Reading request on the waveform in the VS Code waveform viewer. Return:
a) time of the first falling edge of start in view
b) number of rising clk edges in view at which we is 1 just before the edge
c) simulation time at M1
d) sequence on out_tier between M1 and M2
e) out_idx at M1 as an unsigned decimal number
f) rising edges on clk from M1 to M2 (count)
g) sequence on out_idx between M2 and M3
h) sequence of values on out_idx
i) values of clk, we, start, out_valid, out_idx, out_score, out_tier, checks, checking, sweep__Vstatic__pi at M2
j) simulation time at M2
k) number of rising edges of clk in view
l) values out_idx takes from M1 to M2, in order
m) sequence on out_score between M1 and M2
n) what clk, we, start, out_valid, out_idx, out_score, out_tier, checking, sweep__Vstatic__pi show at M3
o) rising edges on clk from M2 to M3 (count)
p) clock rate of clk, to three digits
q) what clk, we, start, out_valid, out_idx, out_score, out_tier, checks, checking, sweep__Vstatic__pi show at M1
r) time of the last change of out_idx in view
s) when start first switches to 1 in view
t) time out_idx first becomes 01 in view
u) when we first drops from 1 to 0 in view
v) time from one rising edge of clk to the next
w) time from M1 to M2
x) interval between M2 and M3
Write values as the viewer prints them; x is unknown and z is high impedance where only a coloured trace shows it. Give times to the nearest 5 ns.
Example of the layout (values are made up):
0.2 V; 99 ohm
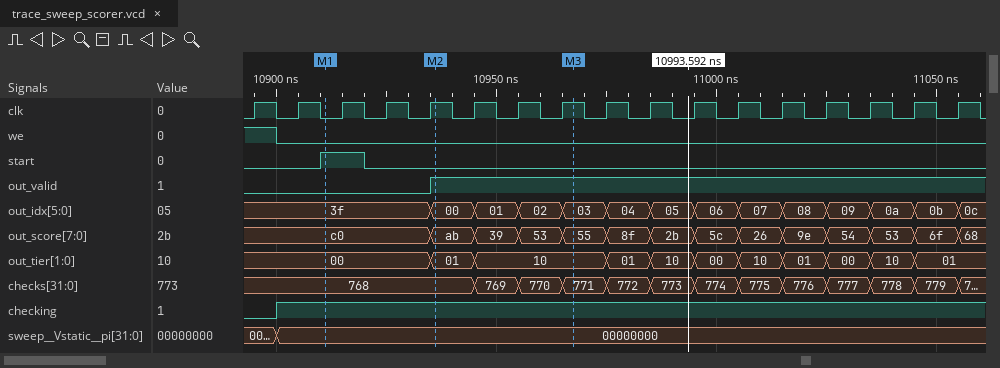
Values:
10920 ns; 1; 10910 ns; 00, 01; 63; 3; 00, 01, 02, 03; 3f, 00, 01, 02, 03, 04, 05, 06, 07, 08, 09, 0a, 0b, 0c; clk=1, we=0, start=0, out_valid=1, out_idx=00, out_score=ab, out_tier=01, checks=768, checking=1, sweep__Vstatic__pi=00000000; 10935 ns; 17; 3f, 00; c0, ab; clk=1, we=0, start=0, out_valid=1, out_idx=03, out_score=55, out_tier=10, checking=1, sweep__Vstatic__pi=00000000; 3; 100 MHz; clk=0, we=0, start=1, out_valid=0, out_idx=3f, out_score=c0, out_tier=00, checks=768, checking=1, sweep__Vstatic__pi=00000000; 11055 ns; 10910 ns; 10945 ns; 10900 ns; 10 ns; 25 ns; 30 ns
